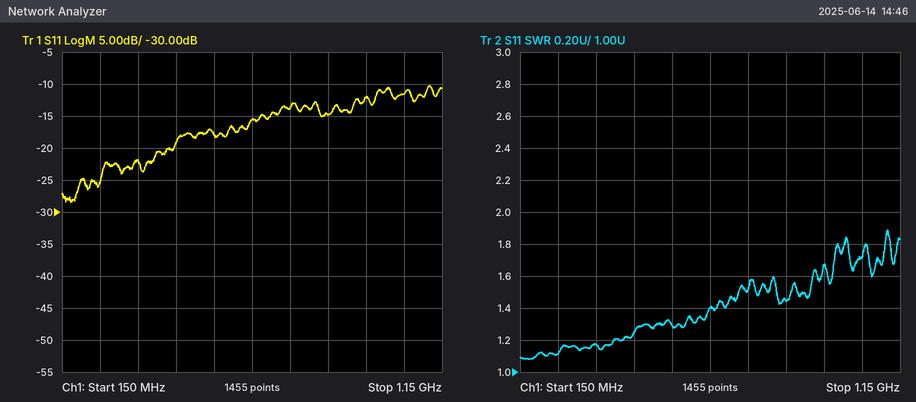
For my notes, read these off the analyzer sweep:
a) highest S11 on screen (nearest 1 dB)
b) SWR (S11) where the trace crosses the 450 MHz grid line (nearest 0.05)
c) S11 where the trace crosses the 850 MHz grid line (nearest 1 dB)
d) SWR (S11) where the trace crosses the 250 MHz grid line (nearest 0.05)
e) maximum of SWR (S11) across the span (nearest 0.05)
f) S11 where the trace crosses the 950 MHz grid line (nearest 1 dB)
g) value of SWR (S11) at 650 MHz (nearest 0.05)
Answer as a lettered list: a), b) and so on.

a) -10 dB
b) 1.25
c) -15 dB
d) 1.10
e) 1.90
f) -12 dB
g) 1.40
